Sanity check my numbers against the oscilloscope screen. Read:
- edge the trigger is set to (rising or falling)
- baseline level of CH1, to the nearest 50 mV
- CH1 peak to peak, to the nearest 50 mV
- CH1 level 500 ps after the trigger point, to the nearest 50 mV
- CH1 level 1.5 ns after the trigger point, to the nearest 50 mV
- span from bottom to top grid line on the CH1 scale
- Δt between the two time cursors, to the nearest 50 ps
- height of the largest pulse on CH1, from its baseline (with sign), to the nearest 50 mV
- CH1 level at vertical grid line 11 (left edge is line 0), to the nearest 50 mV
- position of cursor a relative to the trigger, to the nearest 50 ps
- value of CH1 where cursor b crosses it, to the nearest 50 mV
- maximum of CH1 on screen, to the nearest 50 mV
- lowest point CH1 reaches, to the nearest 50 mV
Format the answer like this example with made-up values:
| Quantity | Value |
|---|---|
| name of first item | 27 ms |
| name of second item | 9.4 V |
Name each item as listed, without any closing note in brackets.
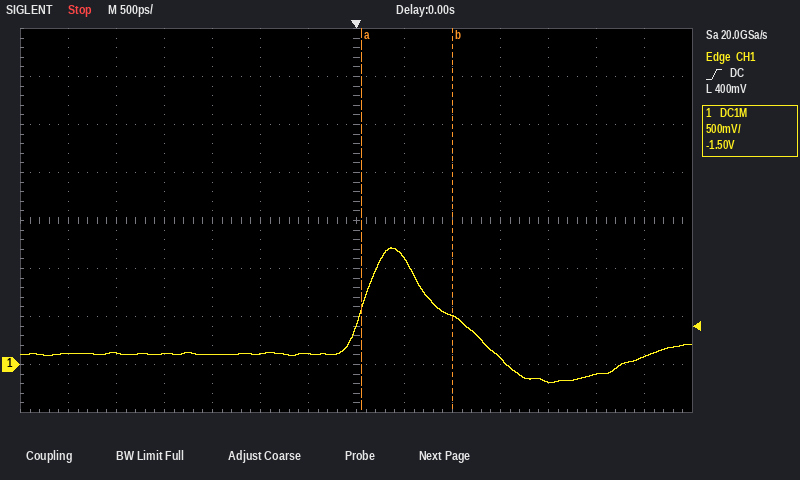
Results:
| Quantity | Value |
|---|---|
| edge the trigger is set to | rising |
| baseline level of CH1, to the nearest 50 mV | 100 mV |
| CH1 peak to peak, to the nearest 50 mV | 1.40 V |
| CH1 level 500 ps after the trigger point, to the nearest 50 mV | 1.10 V |
| CH1 level 1.5 ns after the trigger point, to the nearest 50 mV | 50 mV |
| span from bottom to top grid line on the CH1 scale | 4 V |
| Δt between the two time cursors, to the nearest 50 ps | 950 ps |
| height of the largest pulse on CH1, from its baseline (with sign), to the nearest 50 mV | +1.10 V |
| CH1 level at vertical grid line 11 (left edge is line 0), to the nearest 50 mV | -200 mV |
| position of cursor a relative to the trigger, to the nearest 50 ps | +50 ps |
| value of CH1 where cursor b crosses it, to the nearest 50 mV | 500 mV |
| maximum of CH1 on screen, to the nearest 50 mV | 1.20 V |
| lowest point CH1 reaches, to the nearest 50 mV | -200 mV |
